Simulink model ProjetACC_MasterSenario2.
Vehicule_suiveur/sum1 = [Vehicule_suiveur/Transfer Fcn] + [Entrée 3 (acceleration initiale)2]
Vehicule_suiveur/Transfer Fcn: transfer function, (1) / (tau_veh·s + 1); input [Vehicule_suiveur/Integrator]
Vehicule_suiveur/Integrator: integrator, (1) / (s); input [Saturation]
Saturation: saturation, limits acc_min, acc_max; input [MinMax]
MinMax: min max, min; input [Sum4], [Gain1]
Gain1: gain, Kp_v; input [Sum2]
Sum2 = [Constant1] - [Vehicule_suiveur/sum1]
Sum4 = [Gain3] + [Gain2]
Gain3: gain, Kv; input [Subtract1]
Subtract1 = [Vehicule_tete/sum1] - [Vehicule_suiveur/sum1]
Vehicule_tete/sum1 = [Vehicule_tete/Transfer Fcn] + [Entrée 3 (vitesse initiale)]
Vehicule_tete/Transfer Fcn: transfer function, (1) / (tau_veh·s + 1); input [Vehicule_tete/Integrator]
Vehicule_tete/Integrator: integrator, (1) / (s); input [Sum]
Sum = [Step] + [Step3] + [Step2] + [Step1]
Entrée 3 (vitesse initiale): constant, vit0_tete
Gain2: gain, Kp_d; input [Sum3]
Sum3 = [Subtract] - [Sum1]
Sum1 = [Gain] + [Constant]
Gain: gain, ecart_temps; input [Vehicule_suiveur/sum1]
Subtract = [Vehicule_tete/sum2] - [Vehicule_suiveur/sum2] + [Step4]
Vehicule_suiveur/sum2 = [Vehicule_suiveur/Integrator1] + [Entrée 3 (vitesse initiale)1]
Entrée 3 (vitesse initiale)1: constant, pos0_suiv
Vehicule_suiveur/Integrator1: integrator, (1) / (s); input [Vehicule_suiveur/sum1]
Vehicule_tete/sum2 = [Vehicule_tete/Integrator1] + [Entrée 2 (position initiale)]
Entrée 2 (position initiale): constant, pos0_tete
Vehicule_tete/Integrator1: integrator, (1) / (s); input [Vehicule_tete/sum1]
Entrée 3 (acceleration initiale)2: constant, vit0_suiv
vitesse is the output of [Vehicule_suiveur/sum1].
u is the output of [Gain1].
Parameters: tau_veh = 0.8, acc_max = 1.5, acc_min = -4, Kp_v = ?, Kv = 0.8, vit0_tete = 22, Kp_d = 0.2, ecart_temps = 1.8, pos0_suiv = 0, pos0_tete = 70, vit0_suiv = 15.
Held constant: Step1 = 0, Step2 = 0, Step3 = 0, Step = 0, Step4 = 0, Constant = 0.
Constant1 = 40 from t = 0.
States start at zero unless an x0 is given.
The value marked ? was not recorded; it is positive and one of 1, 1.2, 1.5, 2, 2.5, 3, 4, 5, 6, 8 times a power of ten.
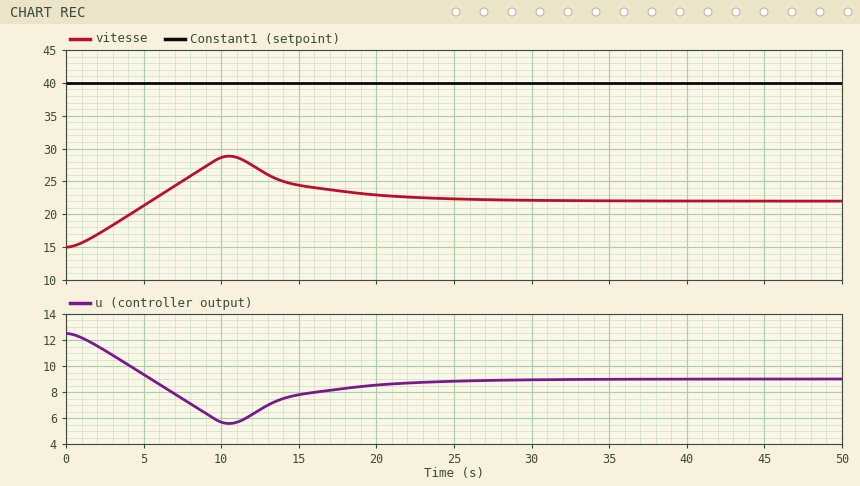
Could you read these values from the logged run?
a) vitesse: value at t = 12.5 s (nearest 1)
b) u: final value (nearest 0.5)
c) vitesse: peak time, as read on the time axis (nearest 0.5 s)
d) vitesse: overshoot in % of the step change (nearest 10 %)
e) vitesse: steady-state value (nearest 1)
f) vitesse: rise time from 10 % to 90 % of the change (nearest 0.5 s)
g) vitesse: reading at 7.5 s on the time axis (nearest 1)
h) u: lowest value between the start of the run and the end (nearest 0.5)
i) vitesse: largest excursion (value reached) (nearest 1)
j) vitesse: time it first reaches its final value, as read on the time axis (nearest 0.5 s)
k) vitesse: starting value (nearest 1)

27
9.0
10.5 s
100 %
22
4.0 s
25
5.5
29
5.5 s
15
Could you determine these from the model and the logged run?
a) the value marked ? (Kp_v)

0.5
